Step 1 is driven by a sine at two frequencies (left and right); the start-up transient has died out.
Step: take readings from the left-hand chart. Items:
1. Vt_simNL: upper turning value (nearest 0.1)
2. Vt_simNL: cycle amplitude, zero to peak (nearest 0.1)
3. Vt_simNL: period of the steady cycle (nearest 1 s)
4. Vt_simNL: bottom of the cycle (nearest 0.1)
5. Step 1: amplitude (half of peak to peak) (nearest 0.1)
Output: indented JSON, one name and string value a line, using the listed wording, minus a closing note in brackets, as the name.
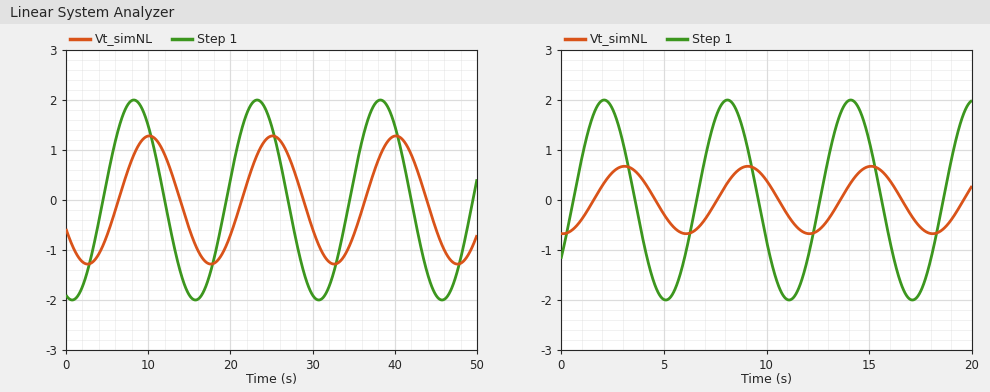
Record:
{
  "Vt_simNL: upper turning value": "1.3",
  "Vt_simNL: cycle amplitude, zero to peak": "1.3",
  "Vt_simNL: period of the steady cycle": "15 s",
  "Vt_simNL: bottom of the cycle": "-1.3",
  "Step 1: amplitude (half of peak to peak)": "2.0"
}
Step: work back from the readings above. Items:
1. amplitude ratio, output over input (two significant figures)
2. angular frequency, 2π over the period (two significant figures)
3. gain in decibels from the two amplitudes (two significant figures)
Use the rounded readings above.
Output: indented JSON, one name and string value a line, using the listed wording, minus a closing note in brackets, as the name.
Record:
{
  "amplitude ratio, output over input": "0.65",
  "angular frequency, 2π over the period": "0.42 rad/s",
  "gain in decibels from the two amplitudes": "-3.7 dB"
}
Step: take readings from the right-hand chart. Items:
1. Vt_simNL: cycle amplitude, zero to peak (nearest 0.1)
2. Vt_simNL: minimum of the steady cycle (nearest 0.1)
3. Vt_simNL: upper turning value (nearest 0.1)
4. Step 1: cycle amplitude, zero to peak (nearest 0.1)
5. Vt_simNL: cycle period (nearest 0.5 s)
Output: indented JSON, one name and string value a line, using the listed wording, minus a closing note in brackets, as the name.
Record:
{
  "Vt_simNL: cycle amplitude, zero to peak": "0.7",
  "Vt_simNL: minimum of the steady cycle": "-0.7",
  "Vt_simNL: upper turning value": "0.7",
  "Step 1: cycle amplitude, zero to peak": "2.0",
  "Vt_simNL: cycle period": "6.0 s"
}
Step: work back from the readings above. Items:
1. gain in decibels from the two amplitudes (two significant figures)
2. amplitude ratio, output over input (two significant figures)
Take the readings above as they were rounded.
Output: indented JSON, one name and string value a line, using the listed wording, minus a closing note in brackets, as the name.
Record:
{
  "gain in decibels from the two amplitudes": "-9.1 dB",
  "amplitude ratio, output over input": "0.35"
}
